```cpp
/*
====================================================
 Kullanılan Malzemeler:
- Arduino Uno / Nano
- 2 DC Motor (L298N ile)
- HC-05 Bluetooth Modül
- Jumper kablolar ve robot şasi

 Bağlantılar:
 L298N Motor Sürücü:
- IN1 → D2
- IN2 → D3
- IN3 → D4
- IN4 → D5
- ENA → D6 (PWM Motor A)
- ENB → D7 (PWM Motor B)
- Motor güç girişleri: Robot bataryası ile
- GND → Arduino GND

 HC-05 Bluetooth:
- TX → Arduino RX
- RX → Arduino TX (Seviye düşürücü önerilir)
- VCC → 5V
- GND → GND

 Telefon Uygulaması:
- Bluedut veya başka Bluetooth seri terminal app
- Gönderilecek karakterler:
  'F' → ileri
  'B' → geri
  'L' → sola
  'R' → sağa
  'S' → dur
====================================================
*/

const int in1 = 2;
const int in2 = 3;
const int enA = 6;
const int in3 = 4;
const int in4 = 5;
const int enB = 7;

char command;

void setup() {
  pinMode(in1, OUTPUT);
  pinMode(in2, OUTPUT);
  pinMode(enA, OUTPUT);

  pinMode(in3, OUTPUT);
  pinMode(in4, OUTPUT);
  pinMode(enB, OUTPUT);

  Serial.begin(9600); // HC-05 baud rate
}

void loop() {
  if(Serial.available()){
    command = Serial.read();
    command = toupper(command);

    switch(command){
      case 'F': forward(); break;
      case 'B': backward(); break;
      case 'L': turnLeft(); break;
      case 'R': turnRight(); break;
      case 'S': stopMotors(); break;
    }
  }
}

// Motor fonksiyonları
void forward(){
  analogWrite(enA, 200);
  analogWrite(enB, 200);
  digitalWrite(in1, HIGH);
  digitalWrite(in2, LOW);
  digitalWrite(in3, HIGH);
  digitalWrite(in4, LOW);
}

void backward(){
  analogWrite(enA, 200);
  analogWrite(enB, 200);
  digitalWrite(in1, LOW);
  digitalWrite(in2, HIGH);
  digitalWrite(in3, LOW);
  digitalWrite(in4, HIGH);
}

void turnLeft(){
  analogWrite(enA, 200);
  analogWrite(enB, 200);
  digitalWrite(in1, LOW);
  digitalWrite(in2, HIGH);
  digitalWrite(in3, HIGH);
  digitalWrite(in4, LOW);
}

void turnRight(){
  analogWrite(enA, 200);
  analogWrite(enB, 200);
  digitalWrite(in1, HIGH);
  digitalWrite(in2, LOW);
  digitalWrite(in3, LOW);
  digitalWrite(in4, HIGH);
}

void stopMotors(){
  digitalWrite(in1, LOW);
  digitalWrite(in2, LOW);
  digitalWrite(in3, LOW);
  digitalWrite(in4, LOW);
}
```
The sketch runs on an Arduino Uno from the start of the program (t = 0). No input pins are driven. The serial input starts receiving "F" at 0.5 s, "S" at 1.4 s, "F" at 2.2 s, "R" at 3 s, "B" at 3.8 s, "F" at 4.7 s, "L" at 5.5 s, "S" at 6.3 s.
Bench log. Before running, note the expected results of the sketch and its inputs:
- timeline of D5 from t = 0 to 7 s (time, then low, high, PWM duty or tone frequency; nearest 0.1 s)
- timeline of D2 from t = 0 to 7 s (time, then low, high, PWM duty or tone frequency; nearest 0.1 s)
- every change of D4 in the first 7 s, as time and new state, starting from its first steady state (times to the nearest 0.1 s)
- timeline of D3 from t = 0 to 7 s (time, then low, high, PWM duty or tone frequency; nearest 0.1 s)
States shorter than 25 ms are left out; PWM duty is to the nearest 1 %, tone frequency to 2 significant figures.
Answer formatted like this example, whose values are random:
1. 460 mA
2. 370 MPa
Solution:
1. 0 s low; 3 s high; 4.7 s low
2. 0 s low; 0.5 s high; 1.4 s low; 2.2 s high; 3.8 s low; 4.7 s high; 5.5 s low
3. 0 s low; 0.5 s high; 1.4 s low; 2.2 s high; 3 s low; 4.7 s high; 6.3 s low
4. 0 s low; 3.8 s high; 4.7 s low; 5.5 s high; 6.3 s low
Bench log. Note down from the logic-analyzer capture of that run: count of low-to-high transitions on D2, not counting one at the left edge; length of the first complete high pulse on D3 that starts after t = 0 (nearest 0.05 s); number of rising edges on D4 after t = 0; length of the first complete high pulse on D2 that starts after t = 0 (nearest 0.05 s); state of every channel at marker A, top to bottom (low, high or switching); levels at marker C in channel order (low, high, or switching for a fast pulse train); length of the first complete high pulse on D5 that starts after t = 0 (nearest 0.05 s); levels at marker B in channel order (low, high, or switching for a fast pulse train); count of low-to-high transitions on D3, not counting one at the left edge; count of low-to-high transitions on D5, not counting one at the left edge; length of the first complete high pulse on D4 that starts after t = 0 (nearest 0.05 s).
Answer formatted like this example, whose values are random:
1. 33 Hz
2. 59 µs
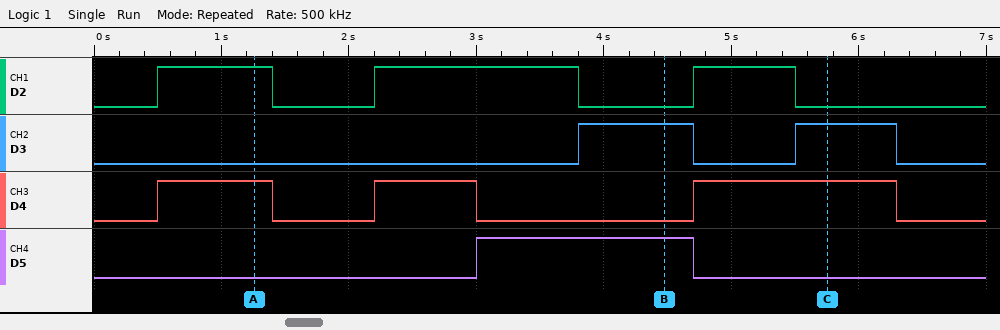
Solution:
1. 3
2. 0.90 s
3. 3
4. 0.90 s
5. D2 high, D3 low, D4 high, D5 low
6. D2 low, D3 high, D4 high, D5 low
7. 1.70 s
8. D2 low, D3 high, D4 low, D5 high
9. 2
10. 1
11. 0.90 s
